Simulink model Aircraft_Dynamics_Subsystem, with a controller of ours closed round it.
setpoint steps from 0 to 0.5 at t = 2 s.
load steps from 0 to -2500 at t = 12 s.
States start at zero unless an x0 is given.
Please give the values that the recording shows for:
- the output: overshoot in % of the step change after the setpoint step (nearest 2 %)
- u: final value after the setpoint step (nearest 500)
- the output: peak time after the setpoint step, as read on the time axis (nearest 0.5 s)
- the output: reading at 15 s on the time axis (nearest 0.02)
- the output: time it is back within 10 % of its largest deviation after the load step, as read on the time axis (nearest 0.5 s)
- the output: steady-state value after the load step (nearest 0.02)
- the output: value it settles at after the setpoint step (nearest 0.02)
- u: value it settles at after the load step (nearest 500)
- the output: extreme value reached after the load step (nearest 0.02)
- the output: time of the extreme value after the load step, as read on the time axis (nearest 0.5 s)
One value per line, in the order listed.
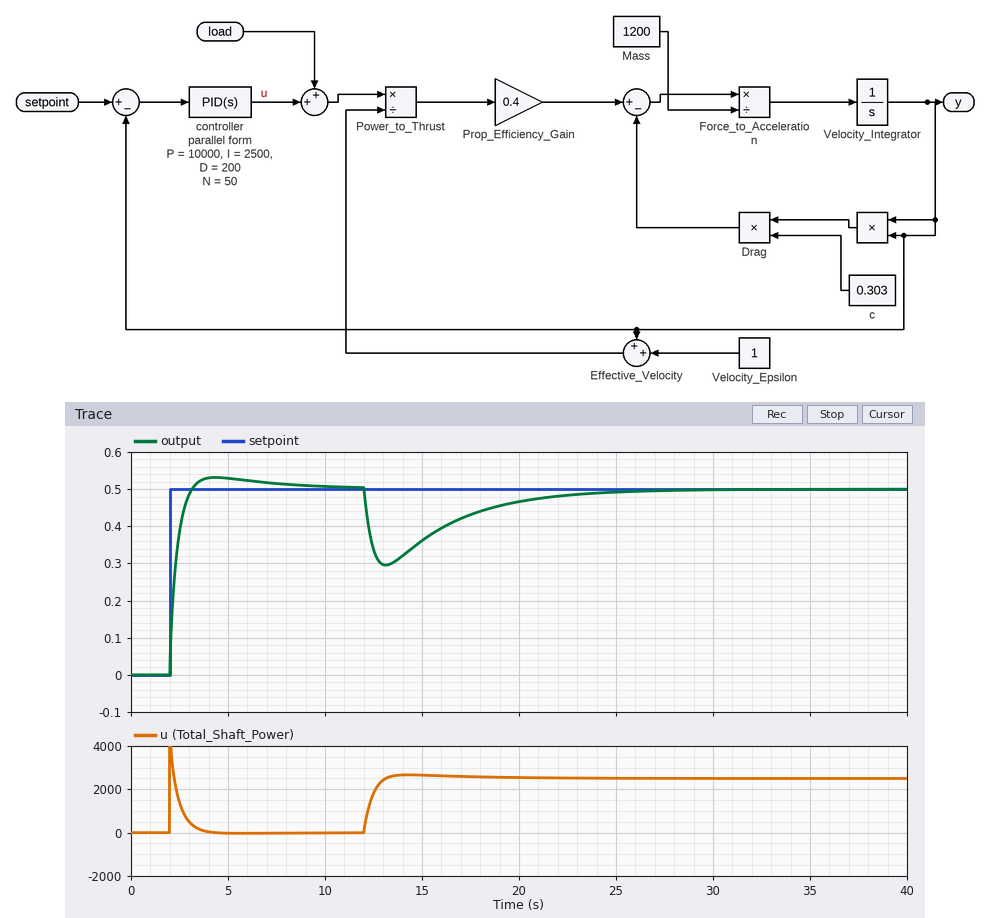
6 %
0
4.5 s
0.36
21.5 s
0.50
0.50
2500
0.30
13.0 s
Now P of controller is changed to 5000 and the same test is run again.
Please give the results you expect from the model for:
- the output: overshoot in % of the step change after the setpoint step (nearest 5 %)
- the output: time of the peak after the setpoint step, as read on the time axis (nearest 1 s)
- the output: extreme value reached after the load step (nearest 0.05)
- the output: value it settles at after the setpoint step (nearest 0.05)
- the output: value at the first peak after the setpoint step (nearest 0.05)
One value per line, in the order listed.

15 %
5 s
0.15
0.50
0.60
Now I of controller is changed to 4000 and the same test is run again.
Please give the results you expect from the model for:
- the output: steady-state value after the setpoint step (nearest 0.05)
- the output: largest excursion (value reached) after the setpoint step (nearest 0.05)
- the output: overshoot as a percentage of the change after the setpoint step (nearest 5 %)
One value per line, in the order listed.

0.50
0.55
10 %
